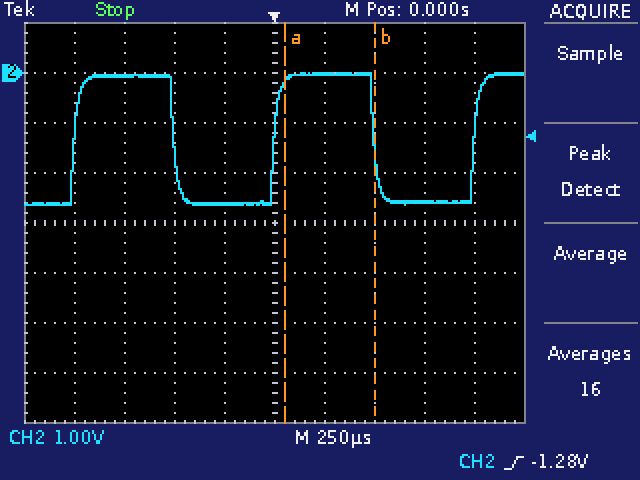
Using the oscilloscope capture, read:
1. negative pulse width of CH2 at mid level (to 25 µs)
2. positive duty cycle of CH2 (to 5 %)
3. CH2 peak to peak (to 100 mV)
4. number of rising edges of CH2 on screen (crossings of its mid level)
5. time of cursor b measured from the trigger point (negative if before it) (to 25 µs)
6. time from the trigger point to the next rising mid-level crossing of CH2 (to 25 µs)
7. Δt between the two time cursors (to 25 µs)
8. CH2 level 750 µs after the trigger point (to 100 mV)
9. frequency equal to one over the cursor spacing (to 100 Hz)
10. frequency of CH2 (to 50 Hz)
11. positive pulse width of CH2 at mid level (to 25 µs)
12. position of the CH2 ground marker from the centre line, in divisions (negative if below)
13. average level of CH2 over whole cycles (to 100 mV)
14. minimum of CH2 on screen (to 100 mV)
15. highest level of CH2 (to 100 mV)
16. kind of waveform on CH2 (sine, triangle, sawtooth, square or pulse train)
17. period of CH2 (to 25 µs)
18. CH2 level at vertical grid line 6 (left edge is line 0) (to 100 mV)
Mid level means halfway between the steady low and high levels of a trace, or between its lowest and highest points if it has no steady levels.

500 µs
50 %
2.6 V
3
+500 µs
1.000 ms
450 µs
-2.6 V
2.2 kHz
1.00 kHz
500 µs
+3.0 div
-1.3 V
-2.6 V
0.0 V
square
1.000 ms
0.0 V
